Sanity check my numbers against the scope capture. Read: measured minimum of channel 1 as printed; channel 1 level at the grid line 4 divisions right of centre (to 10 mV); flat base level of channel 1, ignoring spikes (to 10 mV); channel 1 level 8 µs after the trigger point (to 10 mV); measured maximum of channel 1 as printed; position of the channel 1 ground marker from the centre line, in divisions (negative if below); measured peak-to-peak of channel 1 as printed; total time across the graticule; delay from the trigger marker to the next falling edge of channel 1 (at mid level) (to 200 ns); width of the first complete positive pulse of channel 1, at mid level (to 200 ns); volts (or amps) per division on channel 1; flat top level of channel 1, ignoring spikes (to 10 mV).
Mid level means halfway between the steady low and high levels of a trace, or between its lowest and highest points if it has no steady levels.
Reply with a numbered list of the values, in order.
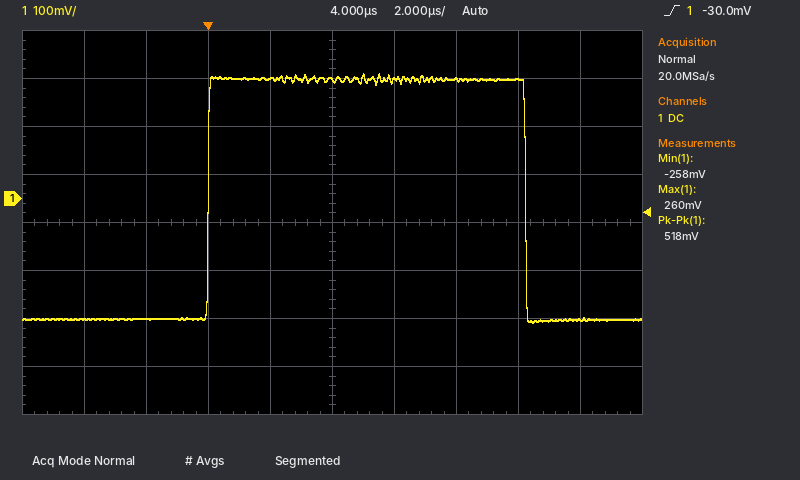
1. -258 mV
2. -250 mV
3. -250 mV
4. 250 mV
5. 260 mV
6. +0.5 div
7. 518 mV
8. 20 µs
9. 10.2 µs
10. 10.2 µs
11. 100 mV
12. 250 mV
